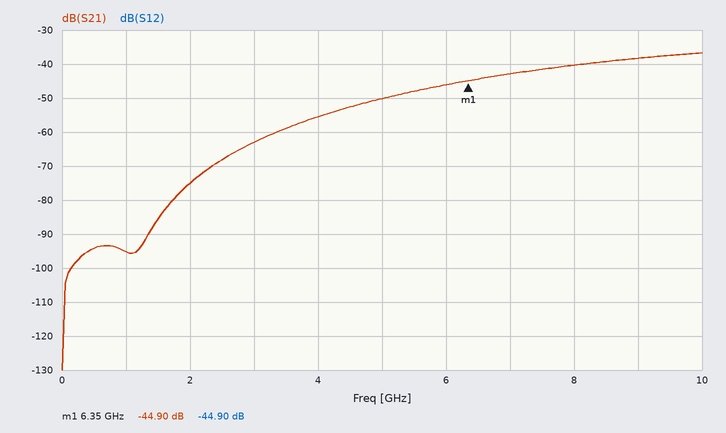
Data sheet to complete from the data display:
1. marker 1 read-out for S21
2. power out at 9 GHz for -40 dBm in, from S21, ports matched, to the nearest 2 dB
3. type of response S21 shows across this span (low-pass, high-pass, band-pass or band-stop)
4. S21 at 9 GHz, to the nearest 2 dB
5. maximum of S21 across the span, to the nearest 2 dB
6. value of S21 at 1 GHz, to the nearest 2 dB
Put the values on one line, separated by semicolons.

-44.90 dB; -78 dBm; high-pass; -38 dB; -36 dB; -96 dB
